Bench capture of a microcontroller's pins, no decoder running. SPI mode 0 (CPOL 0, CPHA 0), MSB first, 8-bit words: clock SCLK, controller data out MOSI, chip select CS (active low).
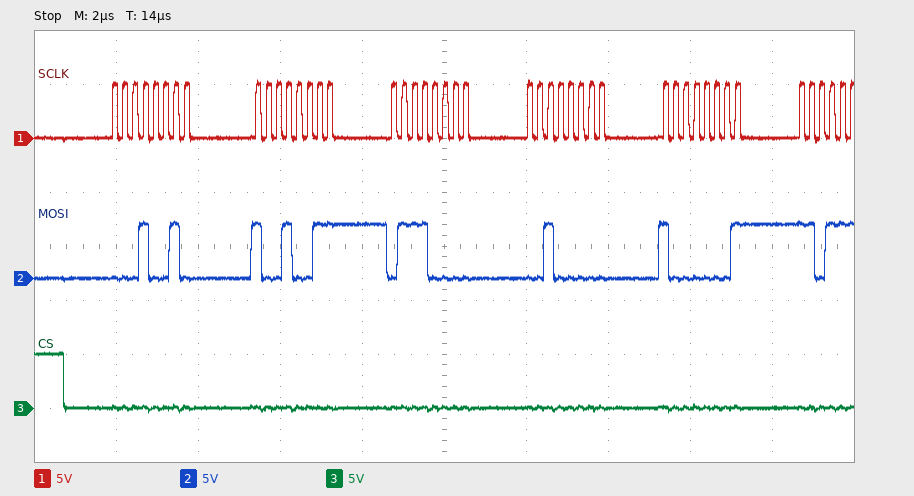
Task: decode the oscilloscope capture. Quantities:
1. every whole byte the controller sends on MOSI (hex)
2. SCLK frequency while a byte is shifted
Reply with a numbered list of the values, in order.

1. 12 93 70 20 81
2. 4 MHz
